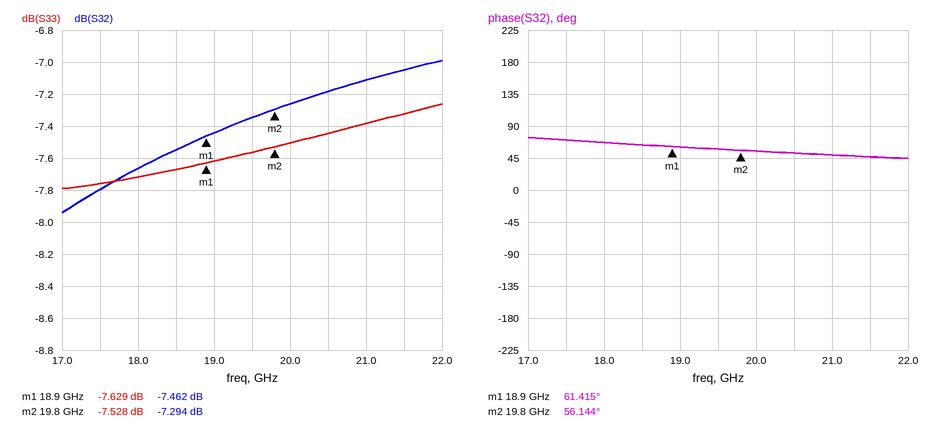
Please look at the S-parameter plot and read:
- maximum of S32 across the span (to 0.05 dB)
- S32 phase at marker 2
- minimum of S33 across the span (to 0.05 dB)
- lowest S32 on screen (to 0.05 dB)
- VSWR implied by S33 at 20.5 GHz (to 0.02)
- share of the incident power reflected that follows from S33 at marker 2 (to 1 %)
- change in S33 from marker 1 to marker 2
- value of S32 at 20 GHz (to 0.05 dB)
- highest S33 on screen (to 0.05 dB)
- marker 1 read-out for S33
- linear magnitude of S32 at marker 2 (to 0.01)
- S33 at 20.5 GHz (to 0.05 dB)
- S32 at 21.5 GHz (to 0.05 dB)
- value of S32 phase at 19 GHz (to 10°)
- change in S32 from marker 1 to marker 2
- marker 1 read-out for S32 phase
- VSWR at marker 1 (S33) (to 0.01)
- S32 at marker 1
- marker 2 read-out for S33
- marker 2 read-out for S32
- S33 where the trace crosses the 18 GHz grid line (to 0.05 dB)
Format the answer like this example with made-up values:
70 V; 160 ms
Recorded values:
-7.00 dB; 56.144°; -7.80 dB; -7.95 dB; 2.48; 18 %; 0.101 dB; -7.25 dB; -7.25 dB; -7.629 dB; 0.43; -7.45 dB; -7.05 dB; 60°; 0.168 dB; 61.415°; 2.42; -7.462 dB; -7.528 dB; -7.294 dB; -7.70 dB
